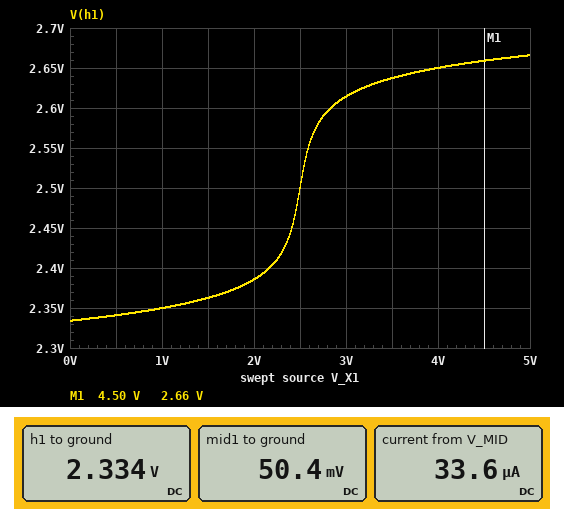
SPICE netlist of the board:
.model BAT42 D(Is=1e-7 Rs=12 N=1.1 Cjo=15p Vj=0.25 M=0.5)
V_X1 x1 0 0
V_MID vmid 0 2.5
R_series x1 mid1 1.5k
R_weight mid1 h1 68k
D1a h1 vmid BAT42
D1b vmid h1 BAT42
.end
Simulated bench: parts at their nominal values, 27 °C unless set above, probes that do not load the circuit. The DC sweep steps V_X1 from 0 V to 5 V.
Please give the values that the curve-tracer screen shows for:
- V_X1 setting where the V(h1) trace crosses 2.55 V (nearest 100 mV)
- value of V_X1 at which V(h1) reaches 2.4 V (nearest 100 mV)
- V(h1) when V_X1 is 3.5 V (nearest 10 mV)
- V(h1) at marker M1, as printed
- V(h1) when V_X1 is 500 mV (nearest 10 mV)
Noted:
2.6 V
2.2 V
2.64 V
2.66 V
2.34 V
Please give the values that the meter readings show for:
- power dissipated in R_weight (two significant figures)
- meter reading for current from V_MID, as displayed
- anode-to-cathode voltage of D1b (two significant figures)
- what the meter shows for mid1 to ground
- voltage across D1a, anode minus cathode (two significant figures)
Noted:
77 µW
33.6 µA
170 mV
50.4 mV
-170 mV
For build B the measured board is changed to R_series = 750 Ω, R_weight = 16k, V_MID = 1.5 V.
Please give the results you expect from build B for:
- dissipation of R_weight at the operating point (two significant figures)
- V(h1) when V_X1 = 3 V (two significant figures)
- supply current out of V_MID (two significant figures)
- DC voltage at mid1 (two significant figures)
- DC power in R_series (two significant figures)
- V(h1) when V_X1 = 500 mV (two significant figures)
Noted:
98 µW
1.7 V
78 µA
59 mV
4.6 µW
1.3 V
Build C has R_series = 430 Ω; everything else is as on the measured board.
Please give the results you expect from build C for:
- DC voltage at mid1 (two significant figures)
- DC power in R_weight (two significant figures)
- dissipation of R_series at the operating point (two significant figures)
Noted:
15 mV
79 µW
500 nW
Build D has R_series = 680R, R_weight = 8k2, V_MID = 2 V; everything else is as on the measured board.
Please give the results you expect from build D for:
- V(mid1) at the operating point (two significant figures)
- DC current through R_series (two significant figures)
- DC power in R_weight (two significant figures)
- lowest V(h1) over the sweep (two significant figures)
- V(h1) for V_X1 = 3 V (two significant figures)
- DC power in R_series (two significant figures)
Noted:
140 mV
200 µA
330 µW
1.8 V
2.2 V
27 µW
